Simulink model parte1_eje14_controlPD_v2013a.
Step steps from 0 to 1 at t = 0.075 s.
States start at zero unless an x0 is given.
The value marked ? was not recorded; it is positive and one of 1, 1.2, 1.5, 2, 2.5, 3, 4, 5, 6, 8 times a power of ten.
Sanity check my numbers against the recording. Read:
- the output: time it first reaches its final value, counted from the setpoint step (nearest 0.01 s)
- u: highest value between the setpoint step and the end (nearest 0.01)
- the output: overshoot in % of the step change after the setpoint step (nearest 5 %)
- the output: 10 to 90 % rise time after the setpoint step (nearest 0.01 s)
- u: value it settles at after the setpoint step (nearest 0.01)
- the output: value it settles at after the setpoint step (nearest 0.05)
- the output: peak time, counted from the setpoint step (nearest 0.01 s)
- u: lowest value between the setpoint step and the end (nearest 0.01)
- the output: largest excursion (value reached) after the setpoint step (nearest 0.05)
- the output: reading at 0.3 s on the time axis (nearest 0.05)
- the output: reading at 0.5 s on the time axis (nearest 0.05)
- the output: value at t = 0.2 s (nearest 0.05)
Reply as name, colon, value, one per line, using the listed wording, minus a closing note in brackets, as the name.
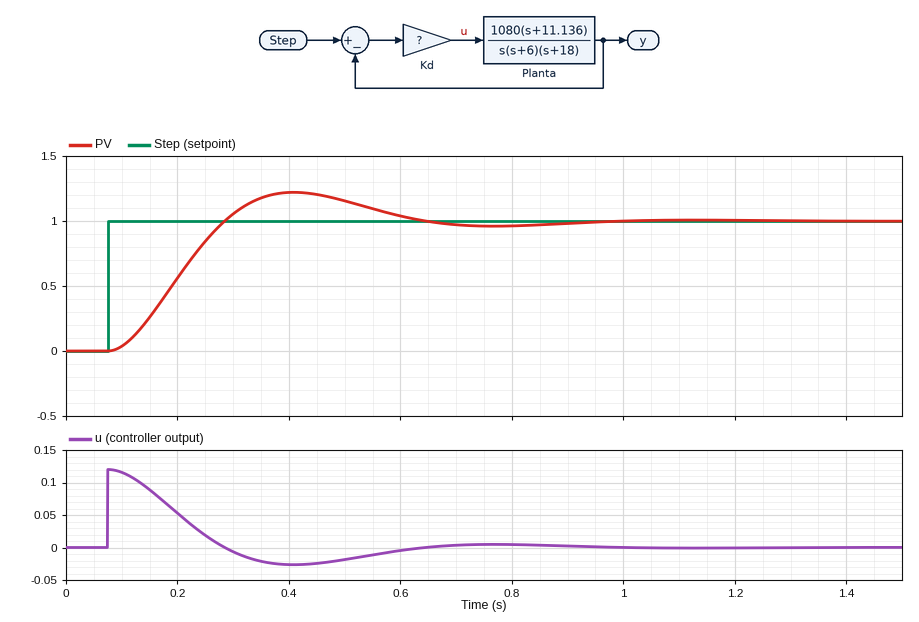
the output: time it first reaches its final value, counted from the setpoint step: 0.21 s
u: highest value between the setpoint step and the end: 0.12
the output: overshoot in % of the step change after the setpoint step: 20 %
the output: 10 to 90 % rise time after the setpoint step: 0.14 s
u: value it settles at after the setpoint step: 0.00
the output: value it settles at after the setpoint step: 1.00
the output: peak time, counted from the setpoint step: 0.33 s
u: lowest value between the setpoint step and the end: -0.03
the output: largest excursion (value reached) after the setpoint step: 1.20
the output: reading at 0.3 s on the time axis: 1.05
the output: reading at 0.5 s on the time axis: 1.15
the output: value at t = 0.2 s: 0.55
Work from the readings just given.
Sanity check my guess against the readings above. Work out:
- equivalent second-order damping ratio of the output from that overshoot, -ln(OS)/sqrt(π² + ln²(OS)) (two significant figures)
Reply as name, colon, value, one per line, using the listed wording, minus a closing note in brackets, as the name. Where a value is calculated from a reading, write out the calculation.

equivalent second-order damping ratio of the output from that overshoot, -ln(OS)/sqrt(π² + ln²(OS)): ln(0.2) = -1.609; 1.609 / sqrt(9.870 + 2.590) = 0.46
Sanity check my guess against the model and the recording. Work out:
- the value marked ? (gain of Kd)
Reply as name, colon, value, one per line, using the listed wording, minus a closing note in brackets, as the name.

the value marked ?: 0.12
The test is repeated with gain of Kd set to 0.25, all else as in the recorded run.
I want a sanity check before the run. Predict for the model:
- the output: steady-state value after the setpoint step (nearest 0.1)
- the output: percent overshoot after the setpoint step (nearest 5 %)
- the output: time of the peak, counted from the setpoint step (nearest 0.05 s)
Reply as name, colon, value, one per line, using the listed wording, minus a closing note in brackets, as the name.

the output: steady-state value after the setpoint step: 1.0
the output: percent overshoot after the setpoint step: 35 %
the output: time of the peak, counted from the setpoint step: 0.20 s
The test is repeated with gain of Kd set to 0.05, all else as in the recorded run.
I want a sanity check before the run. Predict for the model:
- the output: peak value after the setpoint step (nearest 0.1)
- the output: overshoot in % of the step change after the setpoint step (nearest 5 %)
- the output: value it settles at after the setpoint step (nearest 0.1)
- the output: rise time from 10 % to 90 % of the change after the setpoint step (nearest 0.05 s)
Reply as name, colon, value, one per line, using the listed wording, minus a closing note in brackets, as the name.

the output: peak value after the setpoint step: 1.1
the output: overshoot in % of the step change after the setpoint step: 10 %
the output: value it settles at after the setpoint step: 1.0
the output: rise time from 10 % to 90 % of the change after the setpoint step: 0.30 s
